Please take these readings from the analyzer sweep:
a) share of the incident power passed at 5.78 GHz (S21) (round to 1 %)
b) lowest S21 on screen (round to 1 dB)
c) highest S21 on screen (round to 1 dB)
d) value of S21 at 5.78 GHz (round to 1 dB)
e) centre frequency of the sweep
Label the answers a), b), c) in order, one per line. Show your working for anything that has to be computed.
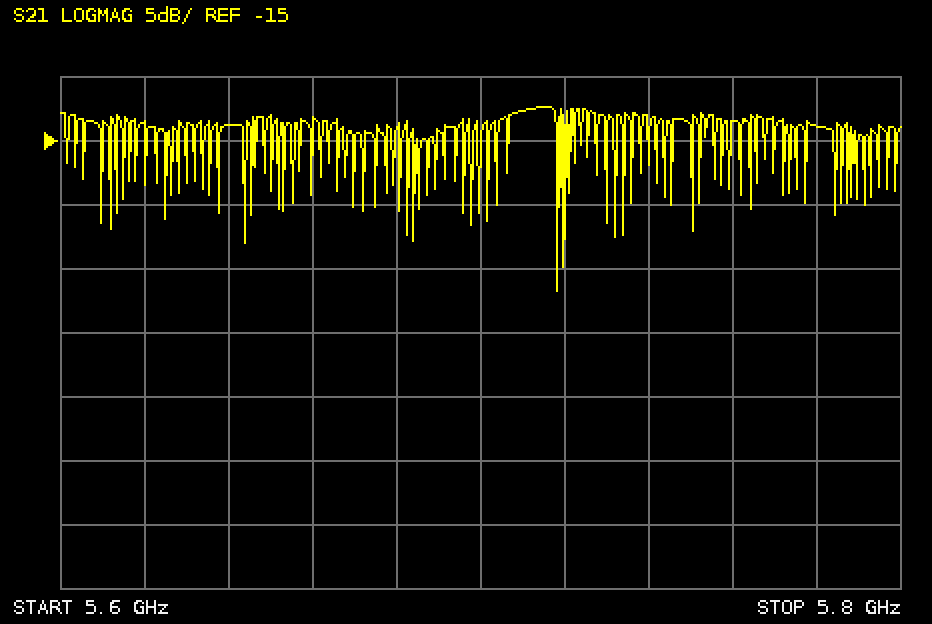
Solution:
a) 10^(-14/10) ≈ 4 %
b) -27 dB
c) -12 dB
d) -14 dB
e) 5.7 GHz
